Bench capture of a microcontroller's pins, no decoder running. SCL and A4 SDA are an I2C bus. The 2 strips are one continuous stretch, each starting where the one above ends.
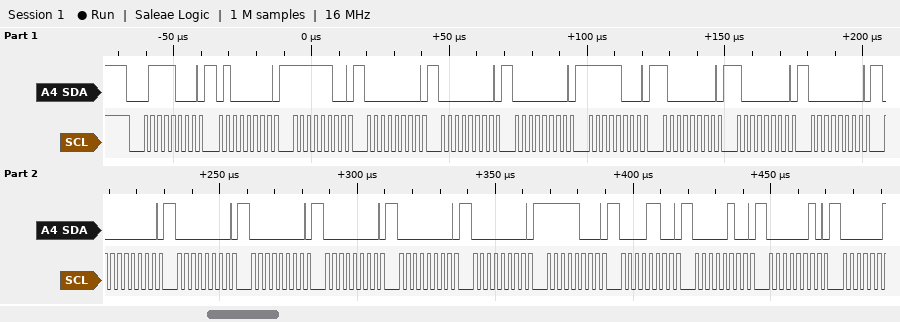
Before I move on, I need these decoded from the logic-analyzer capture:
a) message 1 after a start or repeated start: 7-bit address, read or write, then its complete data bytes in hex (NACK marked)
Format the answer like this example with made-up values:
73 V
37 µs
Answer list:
0x3C write: 40 FC 00 00 00 F8 80 80 00 00 00 00 00 00 00 F8 0C 04 02
